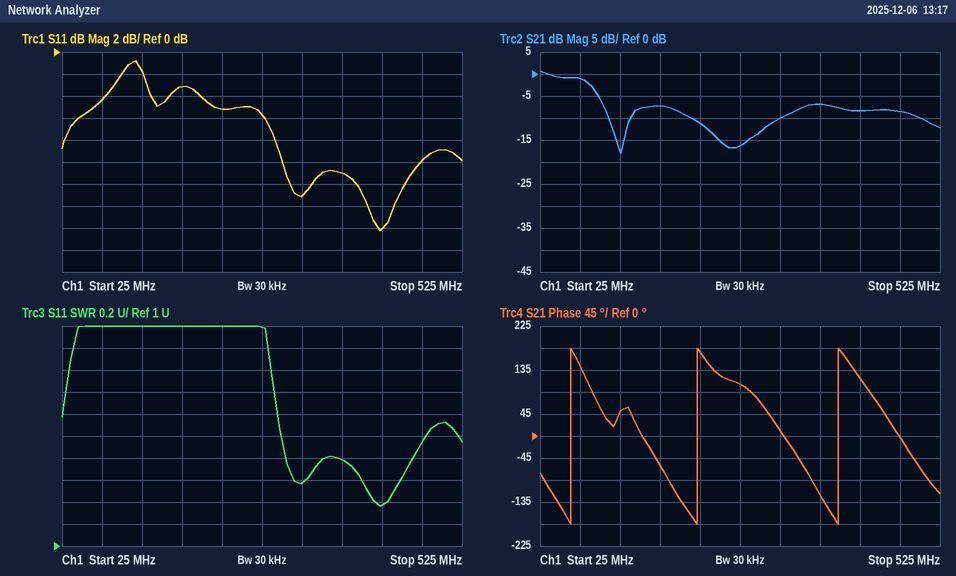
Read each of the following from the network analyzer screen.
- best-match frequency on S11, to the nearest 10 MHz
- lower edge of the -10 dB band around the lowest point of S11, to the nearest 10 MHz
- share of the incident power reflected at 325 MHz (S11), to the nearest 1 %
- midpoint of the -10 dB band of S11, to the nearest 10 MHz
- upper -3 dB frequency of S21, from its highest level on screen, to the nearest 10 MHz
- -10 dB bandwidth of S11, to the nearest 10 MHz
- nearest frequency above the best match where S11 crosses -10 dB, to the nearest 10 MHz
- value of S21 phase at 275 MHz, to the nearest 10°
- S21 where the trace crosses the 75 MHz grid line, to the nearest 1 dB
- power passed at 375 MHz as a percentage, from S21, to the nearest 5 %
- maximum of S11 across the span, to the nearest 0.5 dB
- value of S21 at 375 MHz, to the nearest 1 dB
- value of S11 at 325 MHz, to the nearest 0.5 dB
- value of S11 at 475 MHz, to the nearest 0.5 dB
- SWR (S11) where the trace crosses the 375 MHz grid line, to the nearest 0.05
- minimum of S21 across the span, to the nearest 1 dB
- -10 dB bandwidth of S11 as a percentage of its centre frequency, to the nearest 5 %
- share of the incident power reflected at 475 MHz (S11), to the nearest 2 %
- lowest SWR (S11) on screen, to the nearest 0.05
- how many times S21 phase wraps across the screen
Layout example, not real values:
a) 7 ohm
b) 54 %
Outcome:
a) 420 MHz
b) 300 MHz
c) 5 %
d) 390 MHz
e) 90 MHz
f) 170 MHz
g) 470 MHz
h) 110°
i) -1 dB
j) 20 %
k) -1.0 dB
l) -7 dB
m) -13.0 dB
n) -10.0 dB
o) 1.80
p) -18 dB
q) 45 %
r) 10 %
s) 1.35
t) 3
